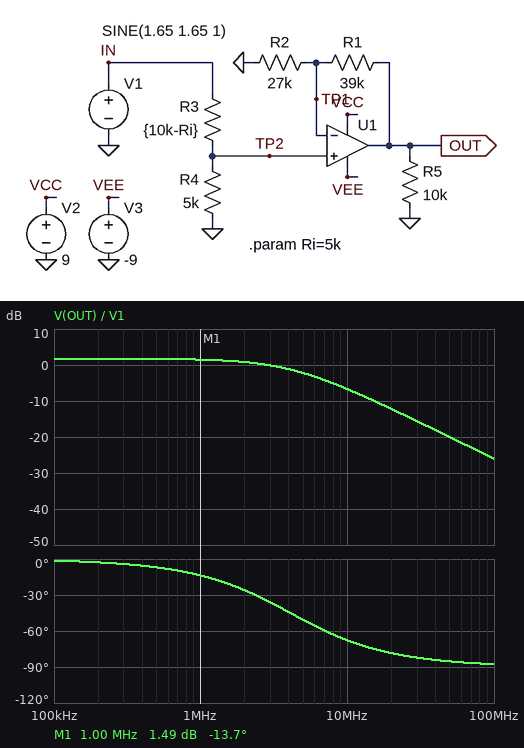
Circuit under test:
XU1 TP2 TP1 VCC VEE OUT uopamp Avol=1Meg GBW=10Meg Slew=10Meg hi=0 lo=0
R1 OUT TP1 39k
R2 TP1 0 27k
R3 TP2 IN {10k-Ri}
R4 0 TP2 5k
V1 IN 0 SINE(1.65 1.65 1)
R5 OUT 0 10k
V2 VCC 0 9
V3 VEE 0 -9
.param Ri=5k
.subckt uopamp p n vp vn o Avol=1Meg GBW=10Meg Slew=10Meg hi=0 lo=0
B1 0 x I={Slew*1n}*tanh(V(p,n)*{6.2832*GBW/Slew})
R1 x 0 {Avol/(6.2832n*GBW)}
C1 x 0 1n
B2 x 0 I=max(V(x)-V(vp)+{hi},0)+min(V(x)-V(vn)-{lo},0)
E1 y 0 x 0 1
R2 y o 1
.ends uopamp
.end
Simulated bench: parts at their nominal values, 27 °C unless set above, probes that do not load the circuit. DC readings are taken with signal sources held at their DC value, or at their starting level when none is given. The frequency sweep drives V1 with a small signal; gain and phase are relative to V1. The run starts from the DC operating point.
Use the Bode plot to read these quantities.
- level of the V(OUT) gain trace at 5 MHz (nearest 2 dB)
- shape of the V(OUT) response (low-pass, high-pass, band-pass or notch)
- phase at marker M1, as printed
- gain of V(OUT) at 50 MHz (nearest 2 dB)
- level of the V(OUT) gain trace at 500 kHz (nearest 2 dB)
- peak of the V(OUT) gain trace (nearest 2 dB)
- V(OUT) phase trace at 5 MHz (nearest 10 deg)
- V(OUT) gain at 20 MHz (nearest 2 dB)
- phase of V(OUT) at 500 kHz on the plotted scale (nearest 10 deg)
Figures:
-2 dB
low-pass
-13.7 deg
-20 dB
2 dB
2 dB
-50 deg
-12 dB
-10 deg
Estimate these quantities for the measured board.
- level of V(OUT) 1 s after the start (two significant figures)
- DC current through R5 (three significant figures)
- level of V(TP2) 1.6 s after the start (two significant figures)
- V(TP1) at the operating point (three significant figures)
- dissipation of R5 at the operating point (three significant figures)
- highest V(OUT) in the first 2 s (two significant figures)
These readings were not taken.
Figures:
2.0 V
202 µA
340 mV
825 mV
407 µW
4.0 V
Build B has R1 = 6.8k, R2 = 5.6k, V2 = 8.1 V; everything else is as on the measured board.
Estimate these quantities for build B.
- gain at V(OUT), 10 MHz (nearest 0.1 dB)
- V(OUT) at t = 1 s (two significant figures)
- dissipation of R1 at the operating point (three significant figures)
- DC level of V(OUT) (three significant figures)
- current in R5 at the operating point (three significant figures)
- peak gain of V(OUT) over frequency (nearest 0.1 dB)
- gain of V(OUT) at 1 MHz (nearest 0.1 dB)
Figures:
-6.8 dB
1.8 V
148 µW
1.83 V
183 µA
0.9 dB
0.7 dB
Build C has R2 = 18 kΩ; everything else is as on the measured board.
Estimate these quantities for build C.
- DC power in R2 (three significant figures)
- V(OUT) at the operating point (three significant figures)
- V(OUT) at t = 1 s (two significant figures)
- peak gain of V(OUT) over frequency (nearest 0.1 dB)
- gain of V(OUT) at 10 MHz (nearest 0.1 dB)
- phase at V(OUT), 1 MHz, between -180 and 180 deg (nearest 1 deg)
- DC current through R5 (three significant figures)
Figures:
37.8 µW
2.61 V
2.6 V
4.0 dB
-6.4 dB
-18 deg
261 µA
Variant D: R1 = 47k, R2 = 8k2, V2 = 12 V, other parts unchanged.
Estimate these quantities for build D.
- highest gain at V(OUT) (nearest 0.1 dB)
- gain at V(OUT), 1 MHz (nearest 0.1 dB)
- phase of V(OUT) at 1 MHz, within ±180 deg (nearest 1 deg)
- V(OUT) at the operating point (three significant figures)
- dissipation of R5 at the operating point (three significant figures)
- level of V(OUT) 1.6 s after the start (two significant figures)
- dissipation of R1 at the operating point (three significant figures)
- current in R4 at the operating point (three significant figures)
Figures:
10.5 dB
8.9 dB
-34 deg
5.55 V
3.08 mW
2.3 V
476 µW
165 µA
